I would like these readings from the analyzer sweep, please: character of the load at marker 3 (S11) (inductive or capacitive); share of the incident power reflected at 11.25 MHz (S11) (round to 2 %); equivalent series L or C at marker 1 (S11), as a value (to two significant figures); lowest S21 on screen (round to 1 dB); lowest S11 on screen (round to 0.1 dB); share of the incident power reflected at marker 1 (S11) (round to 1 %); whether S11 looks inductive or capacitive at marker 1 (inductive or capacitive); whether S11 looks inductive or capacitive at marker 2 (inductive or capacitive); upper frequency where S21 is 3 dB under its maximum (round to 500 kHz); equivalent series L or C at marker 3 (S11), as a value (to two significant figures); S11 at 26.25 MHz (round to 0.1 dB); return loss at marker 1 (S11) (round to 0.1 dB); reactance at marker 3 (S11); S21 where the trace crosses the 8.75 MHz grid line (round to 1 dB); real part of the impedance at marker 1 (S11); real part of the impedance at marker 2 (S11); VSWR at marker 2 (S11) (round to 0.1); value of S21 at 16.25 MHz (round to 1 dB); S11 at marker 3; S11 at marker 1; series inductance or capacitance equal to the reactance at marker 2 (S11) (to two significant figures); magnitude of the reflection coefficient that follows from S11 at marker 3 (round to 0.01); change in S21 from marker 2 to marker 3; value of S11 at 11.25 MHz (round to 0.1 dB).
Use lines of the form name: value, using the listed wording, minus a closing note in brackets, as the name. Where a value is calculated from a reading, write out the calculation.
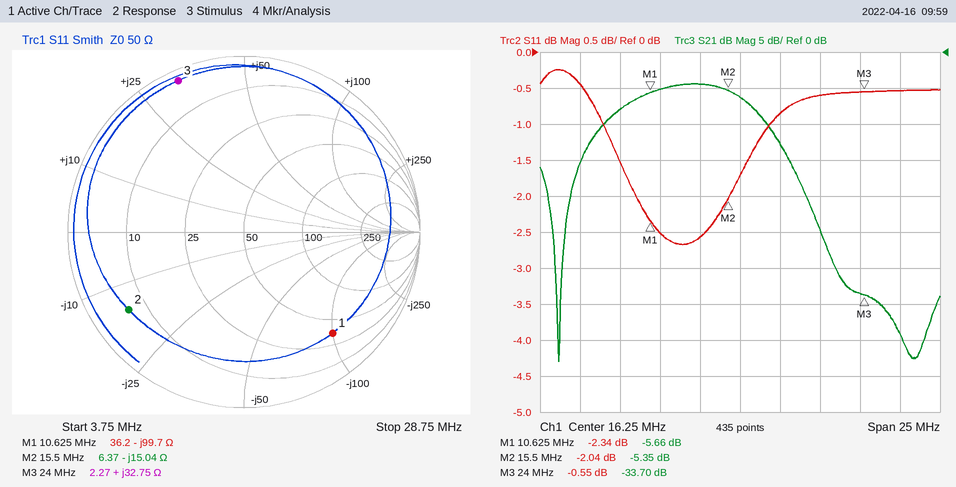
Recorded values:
character of the load at marker 3 (S11): inductive
share of the incident power reflected at 11.25 MHz (S11): 10^(-2.5/10) ≈ 56 %
equivalent series L or C at marker 1 (S11), as a value: C = 1/(2π × 10.625 MHz × 99.7 Ω) ≈ 150 pF
lowest S21 on screen: -43 dB
lowest S11 on screen: -2.7 dB
share of the incident power reflected at marker 1 (S11): 10^(-2.34/10) ≈ 58 %
whether S11 looks inductive or capacitive at marker 1: capacitive
whether S11 looks inductive or capacitive at marker 2: capacitive
upper frequency where S21 is 3 dB under its maximum: 17.0 MHz
equivalent series L or C at marker 3 (S11), as a value: L = 32.75 Ω/(2π × 24 MHz) ≈ 217 nH, so 220 nH to two significant figures
S11 at 26.25 MHz: -0.5 dB
return loss at marker 1 (S11): 2.3 dB
reactance at marker 3: +32.75 Ω
S21 where the trace crosses the 8.75 MHz grid line: -8 dB
real part of the impedance at marker 1: 36.2 Ω
real part of the impedance at marker 2: 6.37 Ω
VSWR at marker 2 (S11): 8.6
value of S21 at 16.25 MHz: -6 dB
S11 at marker 3: -0.55 dB
S11 at marker 1: -2.34 dB
series inductance or capacitance equal to the reactance at marker 2 (S11): C = 1/(2π × 15.5 MHz × 15.04 Ω) ≈ 683 pF, so 680 pF to two significant figures
magnitude of the reflection coefficient that follows from S11 at marker 3: 10^(-0.55/20) ≈ 0.94
change in S21 from marker 2 to marker 3: -33.7 − (-5.35) = -28.35 dB
value of S11 at 11.25 MHz: -2.5 dB
